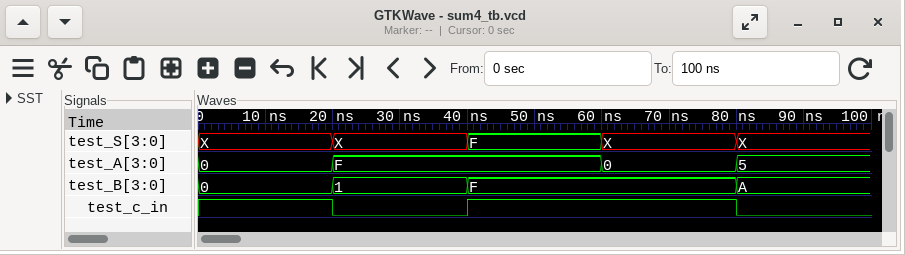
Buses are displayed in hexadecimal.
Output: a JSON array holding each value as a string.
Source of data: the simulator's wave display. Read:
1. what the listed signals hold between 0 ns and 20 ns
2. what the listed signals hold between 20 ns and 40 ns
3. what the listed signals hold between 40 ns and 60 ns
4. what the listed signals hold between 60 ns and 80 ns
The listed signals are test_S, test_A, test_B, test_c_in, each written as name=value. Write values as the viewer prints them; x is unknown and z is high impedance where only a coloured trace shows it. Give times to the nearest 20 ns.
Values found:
["test_S=X, test_A=0, test_B=0, test_c_in=1", "test_S=X, test_A=F, test_B=1, test_c_in=0", "test_S=F, test_A=F, test_B=F, test_c_in=1", "test_S=X, test_A=0, test_B=F, test_c_in=1"]
